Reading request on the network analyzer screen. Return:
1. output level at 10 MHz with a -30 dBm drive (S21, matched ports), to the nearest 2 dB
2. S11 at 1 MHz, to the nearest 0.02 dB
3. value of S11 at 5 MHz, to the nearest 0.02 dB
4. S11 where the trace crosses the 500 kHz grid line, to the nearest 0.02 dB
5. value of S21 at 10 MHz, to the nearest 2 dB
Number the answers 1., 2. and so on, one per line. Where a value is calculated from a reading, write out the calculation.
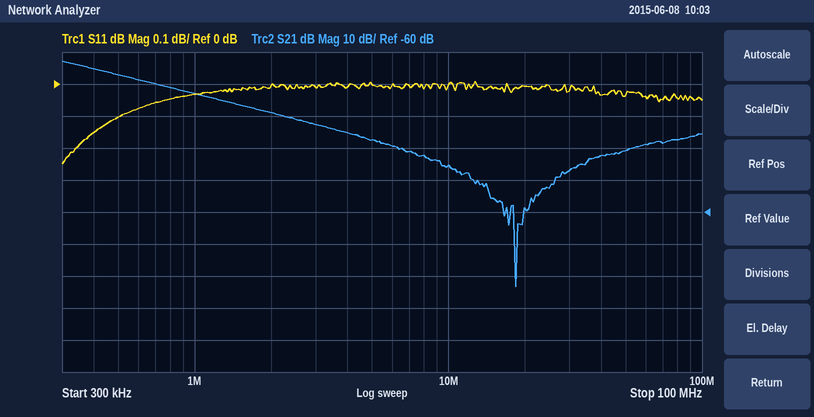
1. -30 dBm + (-46 dB) = -76 dBm
2. -0.04 dB
3. 0.00 dB
4. -0.10 dB
5. -46 dB
